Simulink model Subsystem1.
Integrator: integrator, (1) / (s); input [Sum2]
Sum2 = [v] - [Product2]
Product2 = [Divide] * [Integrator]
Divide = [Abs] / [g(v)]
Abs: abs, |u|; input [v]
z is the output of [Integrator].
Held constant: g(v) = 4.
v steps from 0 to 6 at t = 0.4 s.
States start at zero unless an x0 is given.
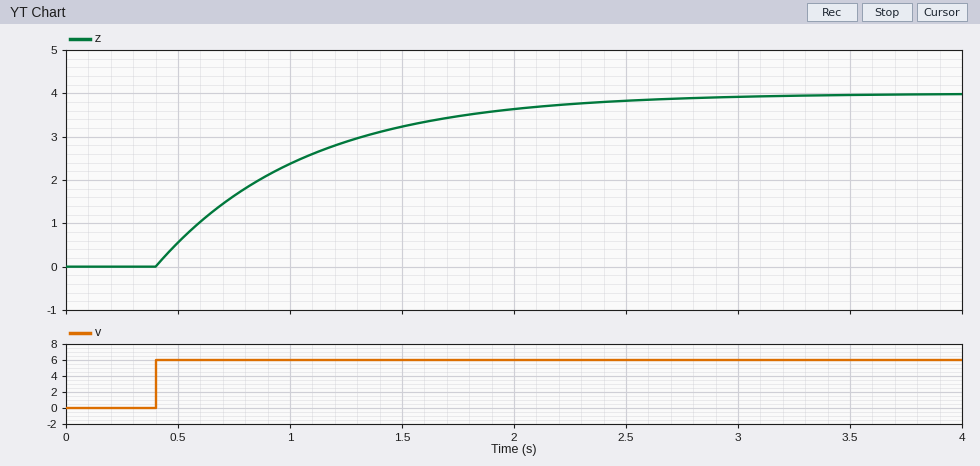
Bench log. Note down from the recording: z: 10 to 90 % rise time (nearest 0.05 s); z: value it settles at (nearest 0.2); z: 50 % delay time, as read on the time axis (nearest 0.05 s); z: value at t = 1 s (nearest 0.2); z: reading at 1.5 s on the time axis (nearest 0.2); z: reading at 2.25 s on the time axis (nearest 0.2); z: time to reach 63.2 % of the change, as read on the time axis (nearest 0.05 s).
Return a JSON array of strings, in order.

["1.45 s", "4.0", "0.85 s", "2.4", "3.2", "3.8", "1.05 s"]
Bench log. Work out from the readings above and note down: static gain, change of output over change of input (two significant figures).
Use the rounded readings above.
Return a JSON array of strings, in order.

["0.67"]
